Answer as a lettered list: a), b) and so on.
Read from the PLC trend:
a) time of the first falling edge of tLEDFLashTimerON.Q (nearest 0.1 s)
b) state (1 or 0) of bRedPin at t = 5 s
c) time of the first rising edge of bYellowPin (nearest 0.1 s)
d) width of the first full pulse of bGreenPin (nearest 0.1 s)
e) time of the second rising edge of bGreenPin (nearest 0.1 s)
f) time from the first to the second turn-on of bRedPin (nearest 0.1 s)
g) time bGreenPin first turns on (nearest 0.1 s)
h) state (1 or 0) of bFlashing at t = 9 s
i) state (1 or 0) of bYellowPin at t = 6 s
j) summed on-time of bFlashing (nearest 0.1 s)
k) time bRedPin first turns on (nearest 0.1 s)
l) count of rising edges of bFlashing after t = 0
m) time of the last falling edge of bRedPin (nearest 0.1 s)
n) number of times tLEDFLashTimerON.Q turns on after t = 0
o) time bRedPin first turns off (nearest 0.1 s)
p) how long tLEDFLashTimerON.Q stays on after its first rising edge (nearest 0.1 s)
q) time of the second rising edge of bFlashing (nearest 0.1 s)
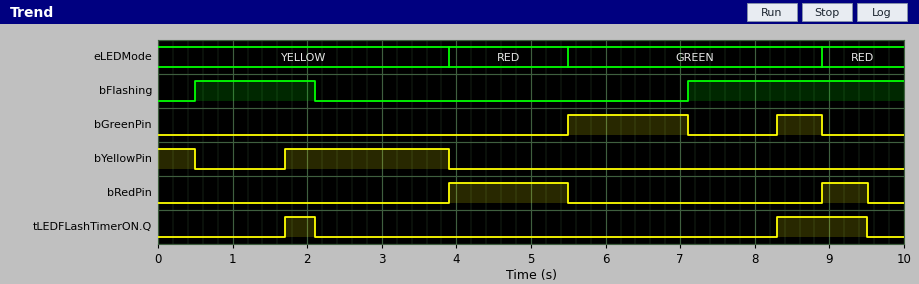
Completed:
a) 2.1 s
b) 1
c) 1.7 s
d) 1.6 s
e) 8.3 s
f) 5.0 s
g) 5.5 s
h) 1
i) 0
j) 4.5 s
k) 3.9 s
l) 2
m) 9.5 s
n) 2
o) 5.5 s
p) 0.4 s
q) 7.1 s
